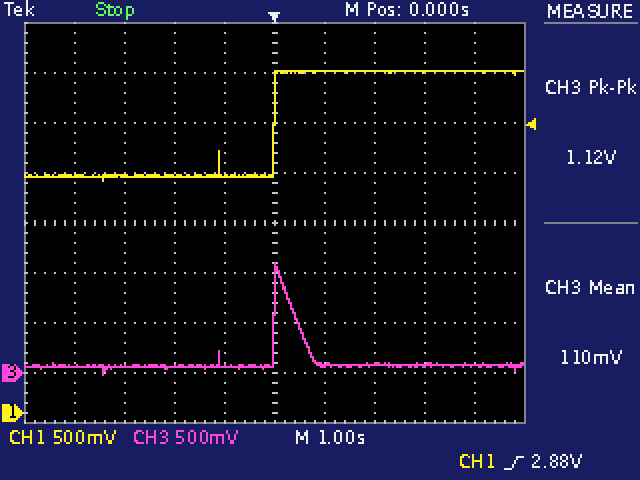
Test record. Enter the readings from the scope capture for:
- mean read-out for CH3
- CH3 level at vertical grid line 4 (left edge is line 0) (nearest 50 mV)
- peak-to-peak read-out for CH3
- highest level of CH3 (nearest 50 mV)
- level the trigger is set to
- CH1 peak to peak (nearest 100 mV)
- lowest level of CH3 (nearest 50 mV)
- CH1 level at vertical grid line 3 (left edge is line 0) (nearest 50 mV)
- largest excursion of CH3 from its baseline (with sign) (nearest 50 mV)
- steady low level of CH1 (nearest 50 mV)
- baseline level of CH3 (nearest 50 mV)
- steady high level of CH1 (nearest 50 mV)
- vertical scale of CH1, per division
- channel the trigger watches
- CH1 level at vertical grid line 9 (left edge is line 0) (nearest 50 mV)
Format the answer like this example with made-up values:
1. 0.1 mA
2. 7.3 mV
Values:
1. 110 mV
2. 50 mV
3. 1.12 V
4. 1.10 V
5. 2.88 V
6. 1.10 V
7. 0 mV
8. 2.35 V
9. +1.05 V
10. 2.35 V
11. 50 mV
12. 3.40 V
13. 500 mV
14. CH1
15. 3.40 V
